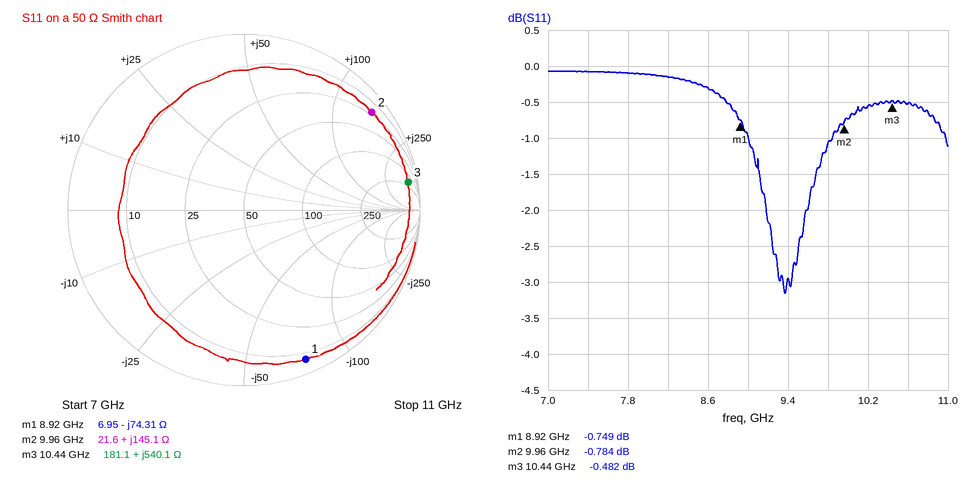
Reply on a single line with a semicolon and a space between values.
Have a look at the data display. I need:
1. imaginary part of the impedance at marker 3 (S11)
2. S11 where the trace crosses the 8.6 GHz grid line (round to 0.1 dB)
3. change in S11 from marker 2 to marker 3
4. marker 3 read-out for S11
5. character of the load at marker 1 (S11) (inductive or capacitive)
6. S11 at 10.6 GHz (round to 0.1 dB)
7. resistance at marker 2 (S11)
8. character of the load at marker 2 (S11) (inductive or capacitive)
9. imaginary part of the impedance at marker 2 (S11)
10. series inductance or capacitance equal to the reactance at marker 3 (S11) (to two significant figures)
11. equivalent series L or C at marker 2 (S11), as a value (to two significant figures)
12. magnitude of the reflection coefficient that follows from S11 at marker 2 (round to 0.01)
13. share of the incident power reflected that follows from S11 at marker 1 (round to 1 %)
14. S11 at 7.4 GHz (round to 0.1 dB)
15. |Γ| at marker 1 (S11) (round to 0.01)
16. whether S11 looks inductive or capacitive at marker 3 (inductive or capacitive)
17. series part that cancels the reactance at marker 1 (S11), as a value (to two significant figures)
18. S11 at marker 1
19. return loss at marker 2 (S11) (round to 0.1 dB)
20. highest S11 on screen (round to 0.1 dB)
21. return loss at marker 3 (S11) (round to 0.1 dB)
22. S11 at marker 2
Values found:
+540.1 Ω; -0.3 dB; 0.302 dB; -0.482 dB; capacitive; -0.5 dB; 21.6 Ω; inductive; +145.1 Ω; 8.2 nH; 2.3 nH; 0.91; 84 %; -0.1 dB; 0.92; inductive; 1.3 nH; -0.749 dB; 0.8 dB; -0.1 dB; 0.5 dB; -0.784 dB
